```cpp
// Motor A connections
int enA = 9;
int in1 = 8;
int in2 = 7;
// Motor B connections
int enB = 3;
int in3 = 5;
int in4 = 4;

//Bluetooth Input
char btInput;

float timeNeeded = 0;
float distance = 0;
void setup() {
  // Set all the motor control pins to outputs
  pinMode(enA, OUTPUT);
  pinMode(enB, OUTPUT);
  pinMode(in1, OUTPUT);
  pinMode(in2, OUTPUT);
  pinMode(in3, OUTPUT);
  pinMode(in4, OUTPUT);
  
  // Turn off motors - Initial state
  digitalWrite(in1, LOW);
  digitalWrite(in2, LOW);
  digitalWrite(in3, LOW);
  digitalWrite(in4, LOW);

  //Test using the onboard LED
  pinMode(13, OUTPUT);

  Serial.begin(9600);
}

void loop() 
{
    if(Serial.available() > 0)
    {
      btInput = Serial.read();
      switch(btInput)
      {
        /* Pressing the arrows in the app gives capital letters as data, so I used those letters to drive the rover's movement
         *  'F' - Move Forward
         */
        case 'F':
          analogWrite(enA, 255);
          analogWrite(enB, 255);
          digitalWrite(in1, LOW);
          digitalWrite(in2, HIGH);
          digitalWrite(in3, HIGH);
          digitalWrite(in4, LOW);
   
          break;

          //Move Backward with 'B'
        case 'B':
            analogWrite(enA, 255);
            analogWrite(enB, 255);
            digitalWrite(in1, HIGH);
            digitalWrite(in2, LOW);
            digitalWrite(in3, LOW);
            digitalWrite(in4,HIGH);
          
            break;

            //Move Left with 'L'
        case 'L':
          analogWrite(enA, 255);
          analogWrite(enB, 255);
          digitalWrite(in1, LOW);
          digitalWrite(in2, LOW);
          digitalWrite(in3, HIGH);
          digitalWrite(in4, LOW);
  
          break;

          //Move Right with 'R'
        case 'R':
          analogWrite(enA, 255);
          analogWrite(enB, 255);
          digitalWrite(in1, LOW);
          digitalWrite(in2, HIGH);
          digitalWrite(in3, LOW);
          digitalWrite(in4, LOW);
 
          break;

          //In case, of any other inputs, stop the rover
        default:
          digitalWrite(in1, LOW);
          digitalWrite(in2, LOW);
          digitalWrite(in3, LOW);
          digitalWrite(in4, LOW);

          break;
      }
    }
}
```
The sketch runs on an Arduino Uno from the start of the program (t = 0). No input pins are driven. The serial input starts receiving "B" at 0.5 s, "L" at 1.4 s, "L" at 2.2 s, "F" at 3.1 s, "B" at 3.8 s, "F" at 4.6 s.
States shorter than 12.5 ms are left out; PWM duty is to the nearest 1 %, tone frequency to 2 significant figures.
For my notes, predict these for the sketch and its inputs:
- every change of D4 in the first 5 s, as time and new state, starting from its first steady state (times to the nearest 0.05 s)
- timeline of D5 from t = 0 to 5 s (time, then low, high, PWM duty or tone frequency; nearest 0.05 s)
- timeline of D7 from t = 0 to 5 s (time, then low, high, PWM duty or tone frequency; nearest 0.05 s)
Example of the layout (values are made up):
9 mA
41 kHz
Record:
0 s low; 0.5 s high; 1.4 s low; 3.8 s high; 4.6 s low
0 s low; 1.4 s high; 3.8 s low; 4.6 s high
0 s low; 3.1 s high; 3.8 s low; 4.6 s high
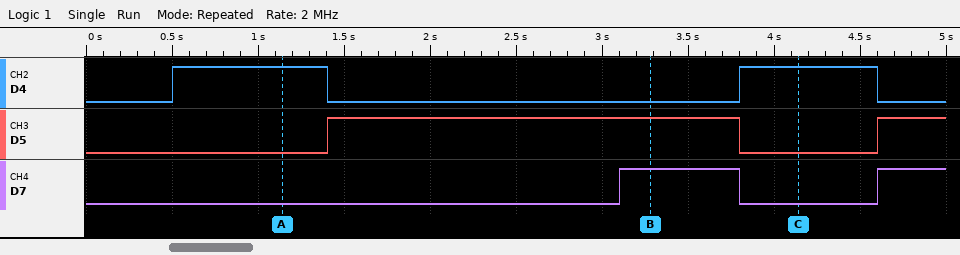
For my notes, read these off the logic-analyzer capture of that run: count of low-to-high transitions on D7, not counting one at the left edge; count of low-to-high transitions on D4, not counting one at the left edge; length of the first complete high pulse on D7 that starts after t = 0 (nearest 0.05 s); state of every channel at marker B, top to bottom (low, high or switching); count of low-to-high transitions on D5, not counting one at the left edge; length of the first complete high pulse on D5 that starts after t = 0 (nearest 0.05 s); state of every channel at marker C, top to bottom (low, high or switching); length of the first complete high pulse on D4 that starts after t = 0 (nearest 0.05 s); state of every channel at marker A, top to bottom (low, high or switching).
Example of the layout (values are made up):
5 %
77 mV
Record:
2
2
0.70 s
D4 low, D5 high, D7 high
2
2.40 s
D4 high, D5 low, D7 low
0.90 s
D4 high, D5 low, D7 low
